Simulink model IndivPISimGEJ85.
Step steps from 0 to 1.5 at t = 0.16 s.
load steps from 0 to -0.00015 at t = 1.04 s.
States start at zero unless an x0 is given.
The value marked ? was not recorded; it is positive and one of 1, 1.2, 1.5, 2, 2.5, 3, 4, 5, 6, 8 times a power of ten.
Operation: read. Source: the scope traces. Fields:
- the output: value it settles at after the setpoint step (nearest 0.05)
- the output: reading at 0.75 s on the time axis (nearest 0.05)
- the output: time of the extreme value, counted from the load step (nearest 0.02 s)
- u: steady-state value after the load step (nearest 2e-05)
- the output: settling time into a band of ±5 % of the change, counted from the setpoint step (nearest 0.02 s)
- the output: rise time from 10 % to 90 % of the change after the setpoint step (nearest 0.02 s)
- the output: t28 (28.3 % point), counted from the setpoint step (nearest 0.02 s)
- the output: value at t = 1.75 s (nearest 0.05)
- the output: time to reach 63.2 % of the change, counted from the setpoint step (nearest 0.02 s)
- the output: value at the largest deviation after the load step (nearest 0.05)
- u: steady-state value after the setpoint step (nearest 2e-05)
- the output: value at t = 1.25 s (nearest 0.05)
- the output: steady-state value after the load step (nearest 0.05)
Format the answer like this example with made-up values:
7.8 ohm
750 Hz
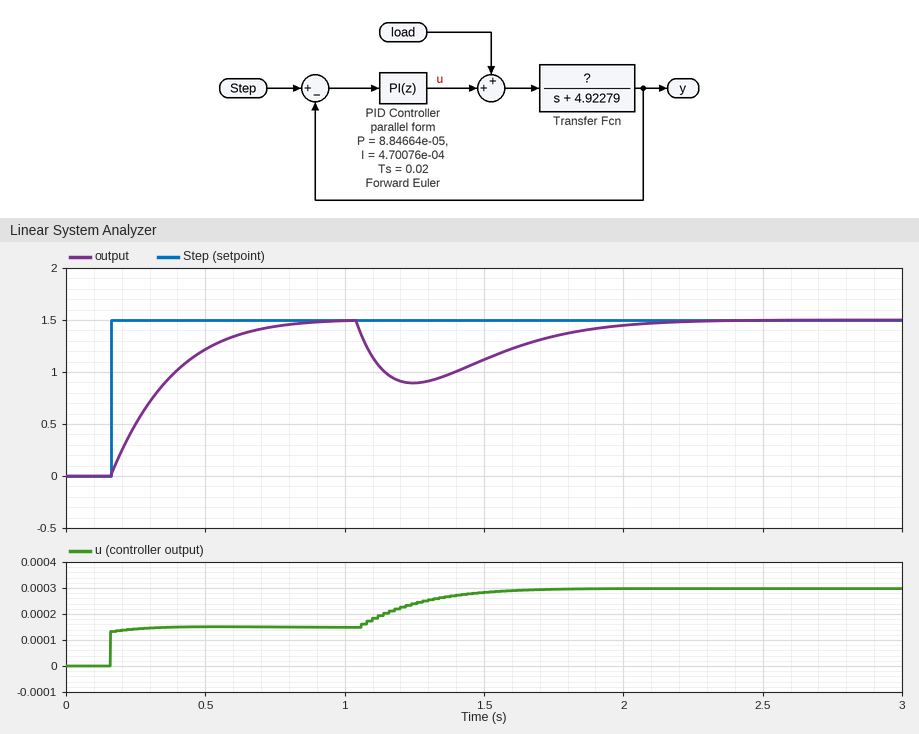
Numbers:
1.50
1.45
0.20 s
0.00030
0.56 s
0.42 s
0.08 s
1.35
0.22 s
0.90
0.00014
0.90
1.50
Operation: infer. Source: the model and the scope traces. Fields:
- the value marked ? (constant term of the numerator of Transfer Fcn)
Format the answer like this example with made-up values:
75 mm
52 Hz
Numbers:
50000
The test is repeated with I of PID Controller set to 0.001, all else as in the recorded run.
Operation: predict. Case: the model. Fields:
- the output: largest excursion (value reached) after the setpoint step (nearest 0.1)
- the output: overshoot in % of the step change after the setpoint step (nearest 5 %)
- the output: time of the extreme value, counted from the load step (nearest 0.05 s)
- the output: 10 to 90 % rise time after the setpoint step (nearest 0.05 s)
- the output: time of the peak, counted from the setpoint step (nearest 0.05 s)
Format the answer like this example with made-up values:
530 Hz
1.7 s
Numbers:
1.7
10 %
0.15 s
0.20 s
0.45 s
